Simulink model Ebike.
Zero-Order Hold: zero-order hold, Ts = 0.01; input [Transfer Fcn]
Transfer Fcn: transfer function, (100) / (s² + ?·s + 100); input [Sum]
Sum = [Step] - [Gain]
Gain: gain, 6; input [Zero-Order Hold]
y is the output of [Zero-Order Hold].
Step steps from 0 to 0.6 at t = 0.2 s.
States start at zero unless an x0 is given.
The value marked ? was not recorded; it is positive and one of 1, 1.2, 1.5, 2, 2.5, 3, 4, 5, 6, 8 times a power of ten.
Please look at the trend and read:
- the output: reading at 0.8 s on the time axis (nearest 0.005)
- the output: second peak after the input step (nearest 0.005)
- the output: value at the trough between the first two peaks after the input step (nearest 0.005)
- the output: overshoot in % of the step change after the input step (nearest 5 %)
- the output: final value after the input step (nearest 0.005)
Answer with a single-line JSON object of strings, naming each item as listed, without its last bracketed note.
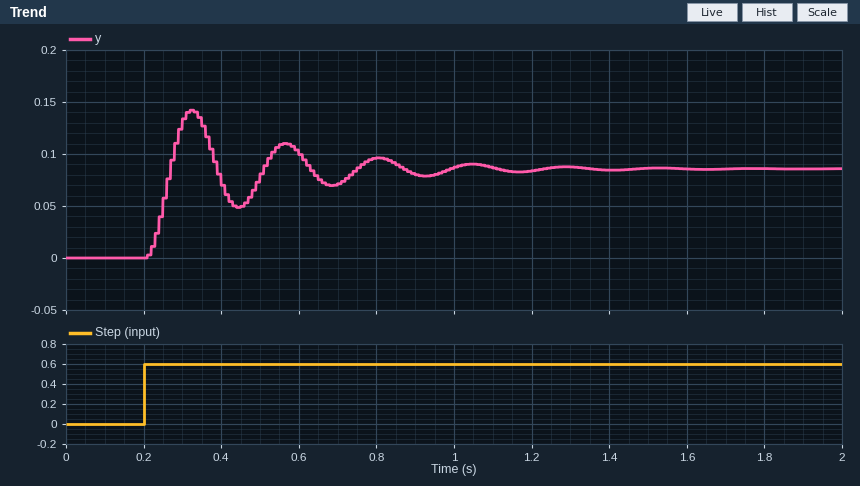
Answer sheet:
{"the output: reading at 0.8 s on the time axis": "0.095", "the output: second peak after the input step": "0.110", "the output: value at the trough between the first two peaks after the input step": "0.050", "the output: overshoot in % of the step change after the input step": "65 %", "the output: final value after the input step": "0.085"}
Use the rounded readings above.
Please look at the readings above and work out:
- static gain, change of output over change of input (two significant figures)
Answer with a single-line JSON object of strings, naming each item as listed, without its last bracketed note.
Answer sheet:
{"static gain, change of output over change of input": "0.14"}
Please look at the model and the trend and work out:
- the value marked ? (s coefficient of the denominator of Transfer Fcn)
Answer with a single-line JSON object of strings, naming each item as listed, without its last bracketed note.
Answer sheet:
{"the value marked ?": "10"}
